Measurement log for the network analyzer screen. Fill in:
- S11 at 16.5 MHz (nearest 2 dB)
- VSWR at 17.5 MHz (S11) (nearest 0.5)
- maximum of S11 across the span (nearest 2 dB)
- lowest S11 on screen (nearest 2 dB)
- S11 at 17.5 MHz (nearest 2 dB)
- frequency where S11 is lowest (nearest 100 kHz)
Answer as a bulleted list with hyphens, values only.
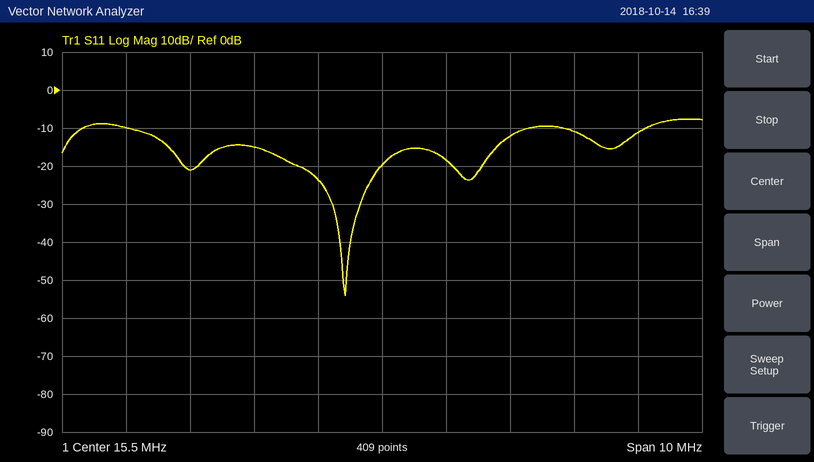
- -18 dB
- 1.5
- -8 dB
- -54 dB
- -12 dB
- 14.9 MHz
